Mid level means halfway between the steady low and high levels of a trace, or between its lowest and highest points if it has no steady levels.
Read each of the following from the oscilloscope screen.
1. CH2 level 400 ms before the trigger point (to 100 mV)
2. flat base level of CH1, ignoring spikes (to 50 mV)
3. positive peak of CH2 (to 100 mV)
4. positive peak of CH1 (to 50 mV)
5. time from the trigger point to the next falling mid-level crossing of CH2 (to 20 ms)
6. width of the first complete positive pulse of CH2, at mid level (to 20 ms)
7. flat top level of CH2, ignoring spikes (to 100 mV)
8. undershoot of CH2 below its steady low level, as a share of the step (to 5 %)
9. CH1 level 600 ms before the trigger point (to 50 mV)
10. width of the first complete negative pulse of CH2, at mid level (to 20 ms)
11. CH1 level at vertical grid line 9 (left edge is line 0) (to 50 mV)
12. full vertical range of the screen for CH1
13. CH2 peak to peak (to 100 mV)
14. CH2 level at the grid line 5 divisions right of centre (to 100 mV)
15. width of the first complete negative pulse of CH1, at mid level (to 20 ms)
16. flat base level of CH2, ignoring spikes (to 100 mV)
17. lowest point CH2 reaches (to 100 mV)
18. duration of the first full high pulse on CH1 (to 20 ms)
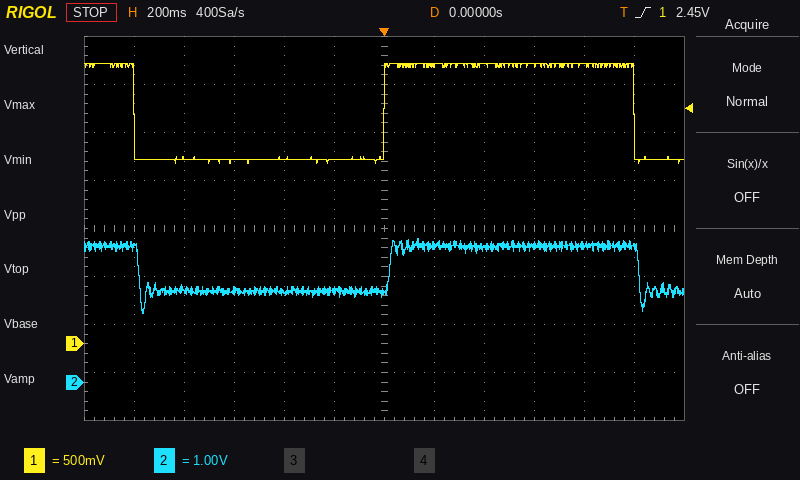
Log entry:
1.9 V
1.90 V
3.0 V
2.90 V
1.02 s
1.00 s
2.8 V
50 %
1.90 V
1.00 s
2.90 V
4 V
1.6 V
2.8 V
1.00 s
1.9 V
1.4 V
1.00 s
